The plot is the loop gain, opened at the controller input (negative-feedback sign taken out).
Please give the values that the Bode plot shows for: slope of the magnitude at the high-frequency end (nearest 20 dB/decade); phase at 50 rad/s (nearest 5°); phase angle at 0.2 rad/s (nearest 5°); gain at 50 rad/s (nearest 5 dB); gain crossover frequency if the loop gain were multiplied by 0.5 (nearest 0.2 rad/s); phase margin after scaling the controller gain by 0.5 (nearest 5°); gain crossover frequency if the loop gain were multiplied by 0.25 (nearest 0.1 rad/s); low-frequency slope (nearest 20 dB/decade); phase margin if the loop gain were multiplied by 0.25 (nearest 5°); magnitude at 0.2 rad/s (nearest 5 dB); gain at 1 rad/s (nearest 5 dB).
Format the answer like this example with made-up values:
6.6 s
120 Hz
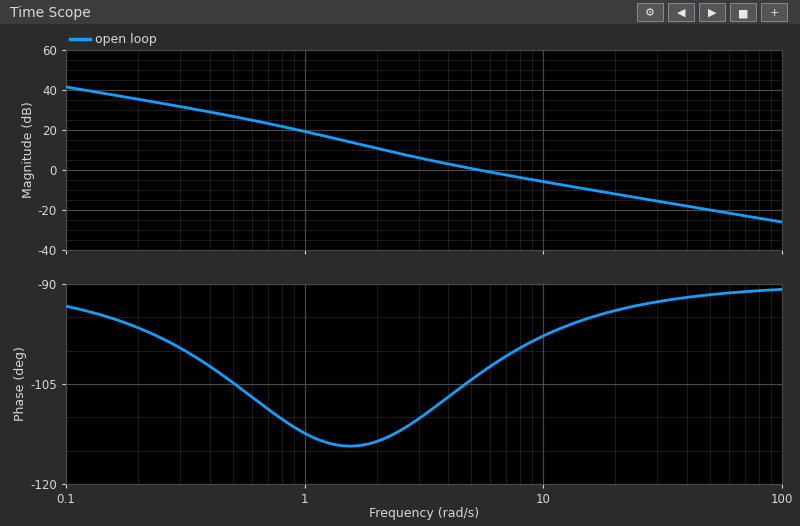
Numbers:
-20 dB/decade
-90°
-95°
-20 dB
3.0 rad/s
70°
1.8 rad/s
-20 dB/decade
65°
35 dB
20 dB
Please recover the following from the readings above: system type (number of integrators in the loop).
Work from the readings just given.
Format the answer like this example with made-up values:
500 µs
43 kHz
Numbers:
1
